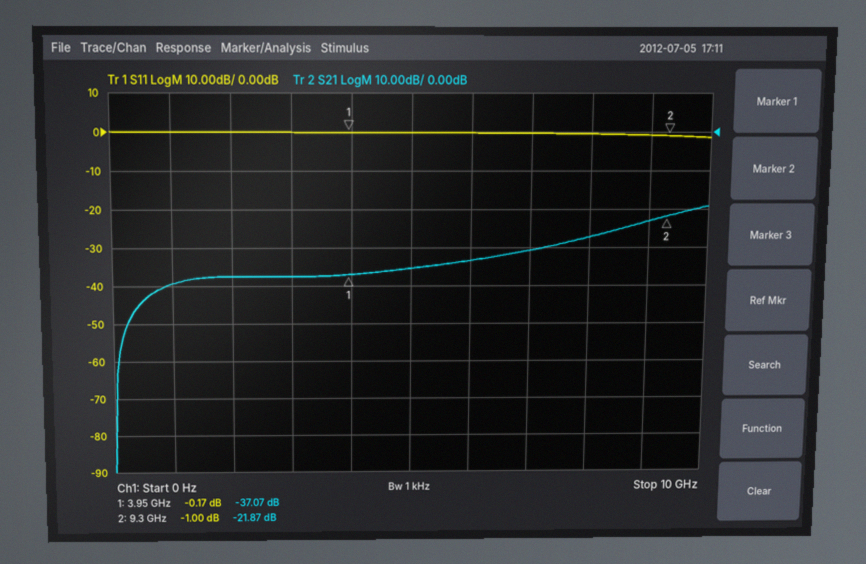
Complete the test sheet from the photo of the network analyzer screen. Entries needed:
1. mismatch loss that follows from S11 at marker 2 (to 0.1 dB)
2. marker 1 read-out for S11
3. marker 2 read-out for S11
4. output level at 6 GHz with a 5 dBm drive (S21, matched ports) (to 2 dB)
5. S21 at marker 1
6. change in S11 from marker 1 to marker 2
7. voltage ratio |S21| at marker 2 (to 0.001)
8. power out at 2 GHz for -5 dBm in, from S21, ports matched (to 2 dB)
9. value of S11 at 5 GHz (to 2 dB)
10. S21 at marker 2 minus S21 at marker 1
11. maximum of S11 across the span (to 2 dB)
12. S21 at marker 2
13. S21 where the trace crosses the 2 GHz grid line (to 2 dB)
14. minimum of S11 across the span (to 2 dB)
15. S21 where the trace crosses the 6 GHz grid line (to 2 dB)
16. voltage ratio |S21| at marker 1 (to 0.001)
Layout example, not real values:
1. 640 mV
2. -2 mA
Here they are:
1. 6.9 dB
2. -0.17 dB
3. -1.00 dB
4. -28 dBm
5. -37.07 dB
6. -0.83 dB
7. 0.081
8. -42 dBm
9. 0 dB
10. 15.20 dB
11. 0 dB
12. -21.87 dB
13. -38 dB
14. -2 dB
15. -34 dB
16. 0.014
